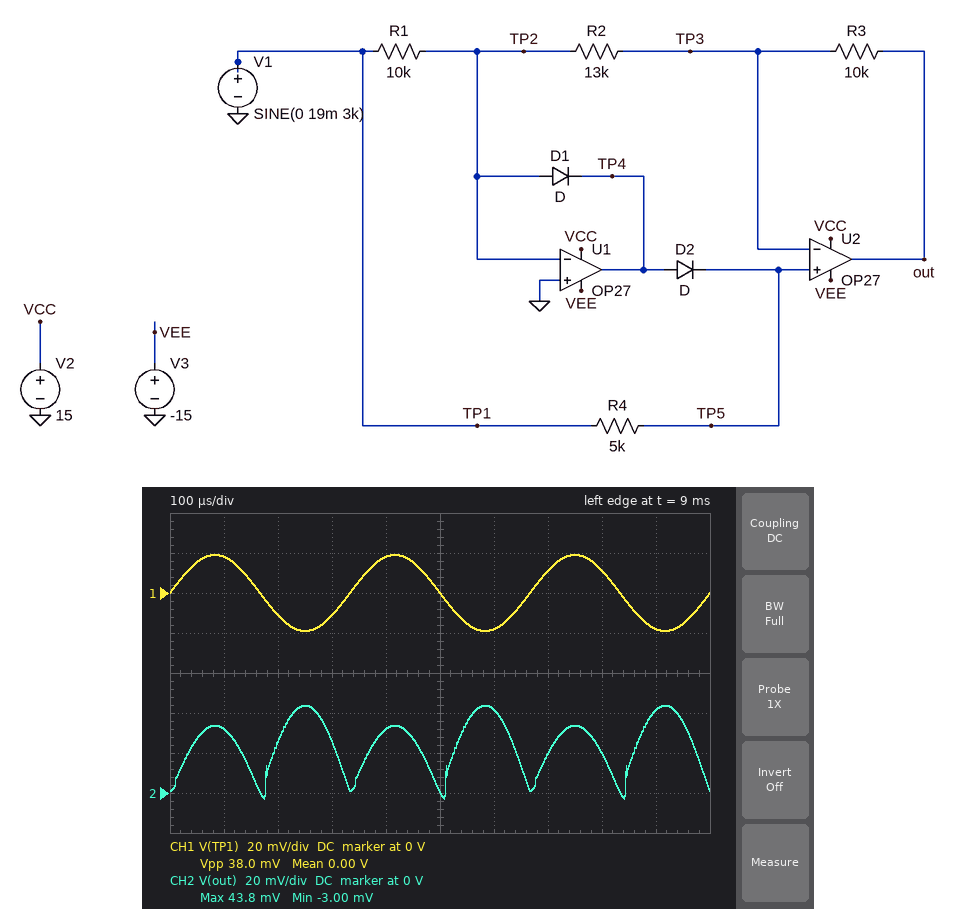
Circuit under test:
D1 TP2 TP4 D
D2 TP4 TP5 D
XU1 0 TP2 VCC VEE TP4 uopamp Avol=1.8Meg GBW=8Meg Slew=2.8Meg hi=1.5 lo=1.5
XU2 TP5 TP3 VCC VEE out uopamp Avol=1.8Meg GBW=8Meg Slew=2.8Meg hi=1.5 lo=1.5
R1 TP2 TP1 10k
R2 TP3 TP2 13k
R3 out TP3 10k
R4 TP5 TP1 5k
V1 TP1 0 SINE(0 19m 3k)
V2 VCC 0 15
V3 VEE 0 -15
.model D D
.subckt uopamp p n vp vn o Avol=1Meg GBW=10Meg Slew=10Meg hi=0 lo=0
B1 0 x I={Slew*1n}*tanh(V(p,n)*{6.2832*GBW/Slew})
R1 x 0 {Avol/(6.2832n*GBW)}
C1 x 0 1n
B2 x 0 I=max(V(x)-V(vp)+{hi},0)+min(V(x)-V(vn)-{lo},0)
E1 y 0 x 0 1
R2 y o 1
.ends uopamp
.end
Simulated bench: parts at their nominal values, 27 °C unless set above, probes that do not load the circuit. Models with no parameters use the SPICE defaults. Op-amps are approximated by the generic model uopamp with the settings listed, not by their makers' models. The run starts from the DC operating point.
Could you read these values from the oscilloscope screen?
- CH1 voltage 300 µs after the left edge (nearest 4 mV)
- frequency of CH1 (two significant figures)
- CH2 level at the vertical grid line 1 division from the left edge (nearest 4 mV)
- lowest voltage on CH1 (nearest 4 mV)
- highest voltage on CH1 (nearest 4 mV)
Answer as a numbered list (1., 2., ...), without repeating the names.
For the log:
1. -12 mV
2. 3.0 kHz
3. 32 mV
4. -20 mV
5. 20 mV
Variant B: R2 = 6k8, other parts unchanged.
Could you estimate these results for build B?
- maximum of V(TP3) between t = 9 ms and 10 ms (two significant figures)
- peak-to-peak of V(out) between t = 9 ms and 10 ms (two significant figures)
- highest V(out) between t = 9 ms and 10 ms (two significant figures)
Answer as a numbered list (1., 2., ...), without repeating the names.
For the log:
1. 19 mV
2. 50 mV
3. 47 mV
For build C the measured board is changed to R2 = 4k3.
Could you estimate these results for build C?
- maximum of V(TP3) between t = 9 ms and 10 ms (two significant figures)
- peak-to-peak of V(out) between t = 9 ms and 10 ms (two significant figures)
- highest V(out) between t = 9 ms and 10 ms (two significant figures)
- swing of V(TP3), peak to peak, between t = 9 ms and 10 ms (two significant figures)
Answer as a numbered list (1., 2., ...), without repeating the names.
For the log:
1. 19 mV
2. 66 mV
3. 63 mV
4. 22 mV
